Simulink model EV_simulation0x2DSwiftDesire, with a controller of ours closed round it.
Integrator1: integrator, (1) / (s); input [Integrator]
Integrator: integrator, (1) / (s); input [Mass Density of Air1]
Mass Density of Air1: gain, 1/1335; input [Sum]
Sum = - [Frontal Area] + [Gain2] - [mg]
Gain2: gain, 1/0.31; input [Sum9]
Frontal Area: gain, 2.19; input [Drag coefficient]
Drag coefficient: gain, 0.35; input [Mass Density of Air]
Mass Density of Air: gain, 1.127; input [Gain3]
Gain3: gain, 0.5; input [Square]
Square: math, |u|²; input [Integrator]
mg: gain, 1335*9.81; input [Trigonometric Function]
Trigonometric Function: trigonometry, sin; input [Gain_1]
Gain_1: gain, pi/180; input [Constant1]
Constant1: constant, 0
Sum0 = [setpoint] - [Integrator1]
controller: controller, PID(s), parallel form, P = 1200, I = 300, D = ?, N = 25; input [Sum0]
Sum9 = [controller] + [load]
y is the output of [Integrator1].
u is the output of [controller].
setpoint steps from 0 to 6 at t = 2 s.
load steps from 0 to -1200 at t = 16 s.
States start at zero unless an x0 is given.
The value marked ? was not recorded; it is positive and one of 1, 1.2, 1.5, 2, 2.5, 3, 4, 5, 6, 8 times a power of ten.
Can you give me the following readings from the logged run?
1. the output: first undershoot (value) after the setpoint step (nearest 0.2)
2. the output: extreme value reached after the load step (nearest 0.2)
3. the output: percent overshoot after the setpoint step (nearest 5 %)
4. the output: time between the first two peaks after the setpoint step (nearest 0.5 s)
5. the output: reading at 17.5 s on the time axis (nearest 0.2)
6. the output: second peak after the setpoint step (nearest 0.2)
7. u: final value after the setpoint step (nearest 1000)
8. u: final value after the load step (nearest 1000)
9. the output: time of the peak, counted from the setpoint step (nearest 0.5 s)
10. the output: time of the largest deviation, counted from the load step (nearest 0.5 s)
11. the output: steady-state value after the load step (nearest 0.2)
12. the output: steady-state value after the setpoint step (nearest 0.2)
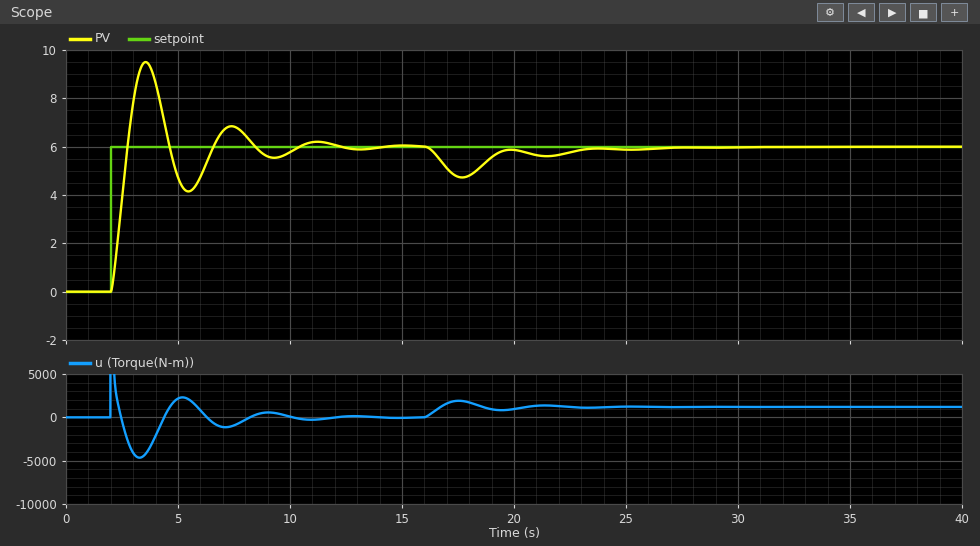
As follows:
4.2
4.8
60 %
4.0 s
4.8
6.8
0
1000
1.5 s
1.5 s
6.0
6.0
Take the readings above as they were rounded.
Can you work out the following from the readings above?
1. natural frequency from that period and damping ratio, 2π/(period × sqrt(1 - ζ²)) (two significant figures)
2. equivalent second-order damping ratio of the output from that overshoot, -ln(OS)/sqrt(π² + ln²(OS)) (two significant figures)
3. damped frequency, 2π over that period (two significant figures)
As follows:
1.6 rad/s
0.16
1.6 rad/s
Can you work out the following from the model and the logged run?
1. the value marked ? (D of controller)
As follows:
400
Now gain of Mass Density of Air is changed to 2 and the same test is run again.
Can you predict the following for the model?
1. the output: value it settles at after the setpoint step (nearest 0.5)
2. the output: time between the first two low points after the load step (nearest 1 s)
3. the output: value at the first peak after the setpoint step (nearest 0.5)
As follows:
6.0
4 s
9.5
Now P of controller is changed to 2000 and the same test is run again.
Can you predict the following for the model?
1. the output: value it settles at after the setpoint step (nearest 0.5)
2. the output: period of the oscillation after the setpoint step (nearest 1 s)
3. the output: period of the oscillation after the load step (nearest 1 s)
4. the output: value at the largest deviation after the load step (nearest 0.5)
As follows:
6.0
3 s
3 s
5.0
